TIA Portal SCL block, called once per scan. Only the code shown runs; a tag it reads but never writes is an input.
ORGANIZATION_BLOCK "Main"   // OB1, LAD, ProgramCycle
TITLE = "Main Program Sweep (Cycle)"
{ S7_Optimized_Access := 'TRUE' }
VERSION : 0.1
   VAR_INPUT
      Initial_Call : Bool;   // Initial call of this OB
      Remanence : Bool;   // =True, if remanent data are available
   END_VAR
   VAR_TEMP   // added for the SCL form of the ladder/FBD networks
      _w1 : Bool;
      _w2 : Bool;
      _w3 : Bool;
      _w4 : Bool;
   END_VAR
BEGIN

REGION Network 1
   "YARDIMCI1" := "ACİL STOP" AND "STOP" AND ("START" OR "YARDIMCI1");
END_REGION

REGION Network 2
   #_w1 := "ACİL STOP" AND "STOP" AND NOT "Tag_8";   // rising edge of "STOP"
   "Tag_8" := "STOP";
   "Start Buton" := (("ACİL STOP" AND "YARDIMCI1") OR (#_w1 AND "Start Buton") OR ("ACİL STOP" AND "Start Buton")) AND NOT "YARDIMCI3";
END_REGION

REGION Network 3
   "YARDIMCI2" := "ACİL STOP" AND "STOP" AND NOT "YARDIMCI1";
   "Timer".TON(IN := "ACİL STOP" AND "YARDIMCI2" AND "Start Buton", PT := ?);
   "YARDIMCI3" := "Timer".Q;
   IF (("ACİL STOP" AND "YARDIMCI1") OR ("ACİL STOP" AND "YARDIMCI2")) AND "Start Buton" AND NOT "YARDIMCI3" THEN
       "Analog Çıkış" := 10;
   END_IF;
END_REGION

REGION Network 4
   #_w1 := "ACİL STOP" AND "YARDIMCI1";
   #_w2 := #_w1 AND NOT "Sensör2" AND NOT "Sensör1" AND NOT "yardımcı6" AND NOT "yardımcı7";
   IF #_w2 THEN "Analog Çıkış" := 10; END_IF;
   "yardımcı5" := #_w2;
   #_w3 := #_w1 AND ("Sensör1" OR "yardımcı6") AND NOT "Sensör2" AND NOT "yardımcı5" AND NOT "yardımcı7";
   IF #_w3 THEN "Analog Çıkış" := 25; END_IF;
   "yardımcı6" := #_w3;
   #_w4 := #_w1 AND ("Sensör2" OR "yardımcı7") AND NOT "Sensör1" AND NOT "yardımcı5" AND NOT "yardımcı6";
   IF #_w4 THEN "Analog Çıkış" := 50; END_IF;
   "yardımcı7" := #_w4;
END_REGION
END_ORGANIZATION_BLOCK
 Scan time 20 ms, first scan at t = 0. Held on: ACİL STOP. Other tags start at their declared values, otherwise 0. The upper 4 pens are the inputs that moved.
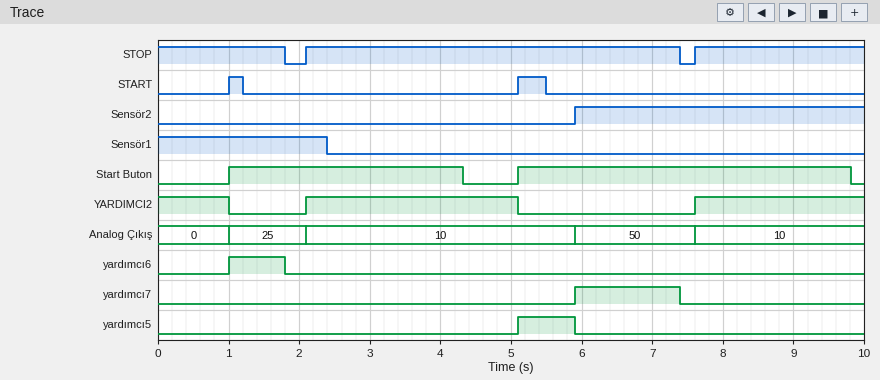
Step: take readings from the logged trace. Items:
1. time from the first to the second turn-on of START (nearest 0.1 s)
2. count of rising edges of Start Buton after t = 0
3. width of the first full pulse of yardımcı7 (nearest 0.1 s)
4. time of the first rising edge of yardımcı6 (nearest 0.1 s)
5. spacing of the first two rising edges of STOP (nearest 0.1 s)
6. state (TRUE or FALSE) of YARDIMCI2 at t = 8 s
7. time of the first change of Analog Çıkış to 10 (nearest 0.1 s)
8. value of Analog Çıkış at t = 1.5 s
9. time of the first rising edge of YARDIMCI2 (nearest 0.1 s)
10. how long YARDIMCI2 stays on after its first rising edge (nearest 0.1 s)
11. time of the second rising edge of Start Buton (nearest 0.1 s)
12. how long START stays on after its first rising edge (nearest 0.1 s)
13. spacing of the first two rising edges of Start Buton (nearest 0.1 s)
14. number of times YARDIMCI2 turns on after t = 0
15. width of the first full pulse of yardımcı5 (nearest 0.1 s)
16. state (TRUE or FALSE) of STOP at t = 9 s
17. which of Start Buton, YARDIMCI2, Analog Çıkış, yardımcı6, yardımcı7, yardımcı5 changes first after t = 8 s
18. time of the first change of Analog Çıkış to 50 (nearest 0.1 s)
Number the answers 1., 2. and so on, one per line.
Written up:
1. 4.1 s
2. 2
3. 1.5 s
4. 1.0 s
5. 5.5 s
6. TRUE
7. 2.1 s
8. 25
9. 2.1 s
10. 3.0 s
11. 5.1 s
12. 0.2 s
13. 4.1 s
14. 2
15. 0.8 s
16. TRUE
17. Start Buton
18. 5.9 s
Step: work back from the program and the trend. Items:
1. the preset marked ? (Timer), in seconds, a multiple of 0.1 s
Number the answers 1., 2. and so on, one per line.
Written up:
1. 2.2 s
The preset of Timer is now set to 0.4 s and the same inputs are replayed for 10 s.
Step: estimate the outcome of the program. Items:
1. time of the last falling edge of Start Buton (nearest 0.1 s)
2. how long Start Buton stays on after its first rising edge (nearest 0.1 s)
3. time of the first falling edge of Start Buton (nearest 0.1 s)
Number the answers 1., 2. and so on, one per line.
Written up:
1. 8.0 s
2. 1.5 s
3. 2.5 s
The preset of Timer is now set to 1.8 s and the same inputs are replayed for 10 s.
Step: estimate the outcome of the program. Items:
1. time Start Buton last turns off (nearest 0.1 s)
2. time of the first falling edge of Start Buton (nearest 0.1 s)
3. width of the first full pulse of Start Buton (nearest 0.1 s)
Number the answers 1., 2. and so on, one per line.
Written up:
1. 9.4 s
2. 3.9 s
3. 2.9 s
